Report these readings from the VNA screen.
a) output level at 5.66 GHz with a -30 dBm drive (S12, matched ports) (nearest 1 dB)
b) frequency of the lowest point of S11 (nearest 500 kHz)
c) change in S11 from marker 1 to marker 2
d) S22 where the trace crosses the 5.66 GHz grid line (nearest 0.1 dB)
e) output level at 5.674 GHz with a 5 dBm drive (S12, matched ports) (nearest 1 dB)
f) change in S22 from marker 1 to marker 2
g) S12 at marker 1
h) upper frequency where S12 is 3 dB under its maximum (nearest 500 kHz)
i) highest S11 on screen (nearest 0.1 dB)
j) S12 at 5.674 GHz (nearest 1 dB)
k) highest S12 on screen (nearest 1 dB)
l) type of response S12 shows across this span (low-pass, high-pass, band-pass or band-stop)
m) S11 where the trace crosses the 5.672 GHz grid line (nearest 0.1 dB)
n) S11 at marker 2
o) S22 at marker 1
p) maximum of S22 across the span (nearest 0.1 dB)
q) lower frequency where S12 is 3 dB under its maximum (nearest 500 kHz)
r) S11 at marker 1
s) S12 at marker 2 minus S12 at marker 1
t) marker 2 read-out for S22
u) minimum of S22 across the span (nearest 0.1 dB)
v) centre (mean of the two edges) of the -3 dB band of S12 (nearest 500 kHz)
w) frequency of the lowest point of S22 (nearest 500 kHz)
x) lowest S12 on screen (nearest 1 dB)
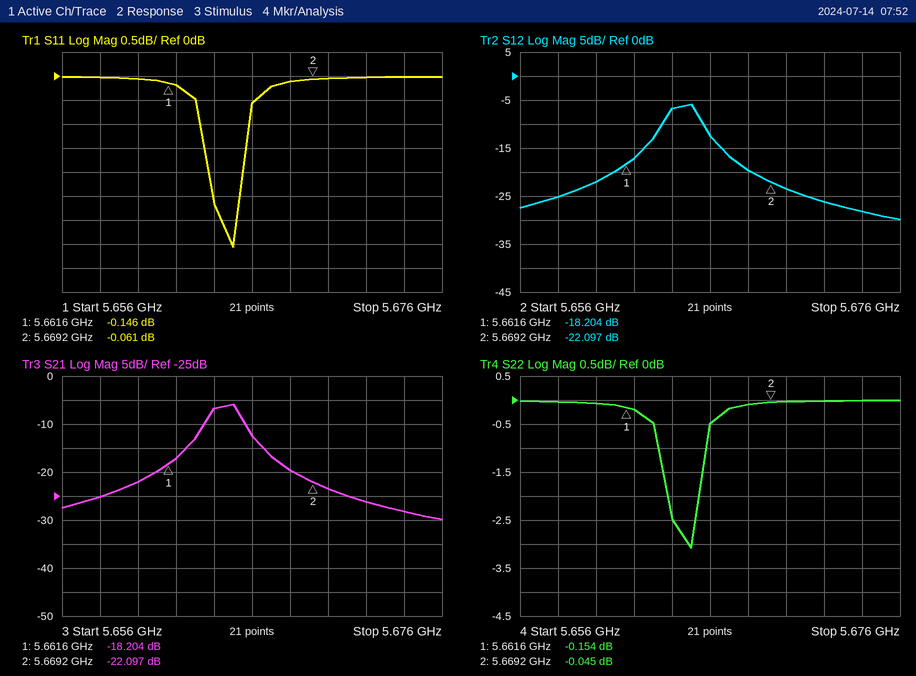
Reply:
-52 dBm
5.6650 GHz
0.085 dB
-0.1 dB
-23 dBm
0.109 dB
-18.204 dB
5.6655 GHz
0.0 dB
-28 dB
-6 dB
band-pass
0.0 dB
-0.061 dB
-0.154 dB
0.0 dB
5.6635 GHz
-0.146 dB
-3.893 dB
-0.045 dB
-3.1 dB
5.6645 GHz
5.6650 GHz
-30 dB
